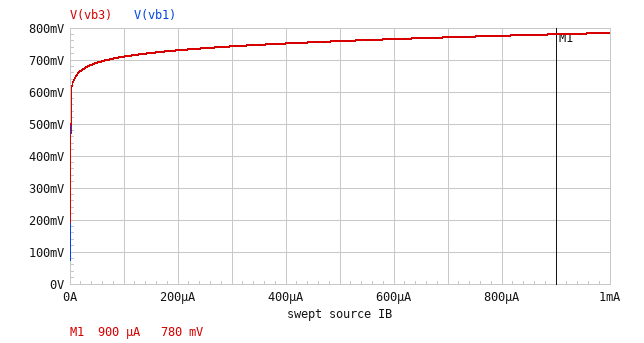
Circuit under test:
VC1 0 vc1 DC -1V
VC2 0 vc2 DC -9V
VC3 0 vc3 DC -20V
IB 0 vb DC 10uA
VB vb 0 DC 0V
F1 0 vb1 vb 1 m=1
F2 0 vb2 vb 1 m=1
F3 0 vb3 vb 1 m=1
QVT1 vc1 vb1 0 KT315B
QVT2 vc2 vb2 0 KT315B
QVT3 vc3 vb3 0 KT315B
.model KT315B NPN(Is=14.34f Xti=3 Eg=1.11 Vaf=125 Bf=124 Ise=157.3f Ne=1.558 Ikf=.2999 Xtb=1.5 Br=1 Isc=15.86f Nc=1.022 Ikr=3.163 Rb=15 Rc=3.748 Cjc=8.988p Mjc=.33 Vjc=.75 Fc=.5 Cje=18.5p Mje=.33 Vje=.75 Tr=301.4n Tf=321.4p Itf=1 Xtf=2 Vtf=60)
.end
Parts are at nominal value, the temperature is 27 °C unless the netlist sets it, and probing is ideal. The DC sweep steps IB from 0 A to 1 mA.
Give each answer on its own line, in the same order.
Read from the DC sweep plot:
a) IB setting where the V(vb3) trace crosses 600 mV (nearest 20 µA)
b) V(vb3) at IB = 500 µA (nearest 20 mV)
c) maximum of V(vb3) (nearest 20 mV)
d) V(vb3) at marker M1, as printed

0 A
760 mV
780 mV
780 mV
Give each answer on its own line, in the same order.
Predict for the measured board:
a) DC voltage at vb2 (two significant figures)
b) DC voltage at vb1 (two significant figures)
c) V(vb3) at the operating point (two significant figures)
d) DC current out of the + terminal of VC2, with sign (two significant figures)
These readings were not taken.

650 mV
650 mV
650 mV
-1.1 mA
